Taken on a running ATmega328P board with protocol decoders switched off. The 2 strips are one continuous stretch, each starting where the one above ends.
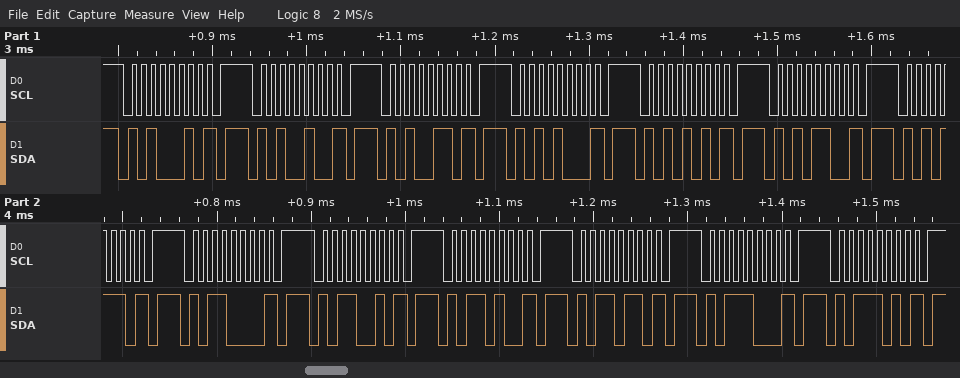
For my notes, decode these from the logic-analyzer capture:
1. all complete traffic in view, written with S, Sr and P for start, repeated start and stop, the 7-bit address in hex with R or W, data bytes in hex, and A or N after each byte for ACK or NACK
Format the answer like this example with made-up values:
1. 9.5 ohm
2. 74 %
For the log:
1. S 51W N P S 52W N P S 53W N P S 54W N P S 55W N P S 56W N P S 57W N P S 58W N P S 59W N P S 5AW N P S 5BW N P S 5CW N P S 5DW N P
